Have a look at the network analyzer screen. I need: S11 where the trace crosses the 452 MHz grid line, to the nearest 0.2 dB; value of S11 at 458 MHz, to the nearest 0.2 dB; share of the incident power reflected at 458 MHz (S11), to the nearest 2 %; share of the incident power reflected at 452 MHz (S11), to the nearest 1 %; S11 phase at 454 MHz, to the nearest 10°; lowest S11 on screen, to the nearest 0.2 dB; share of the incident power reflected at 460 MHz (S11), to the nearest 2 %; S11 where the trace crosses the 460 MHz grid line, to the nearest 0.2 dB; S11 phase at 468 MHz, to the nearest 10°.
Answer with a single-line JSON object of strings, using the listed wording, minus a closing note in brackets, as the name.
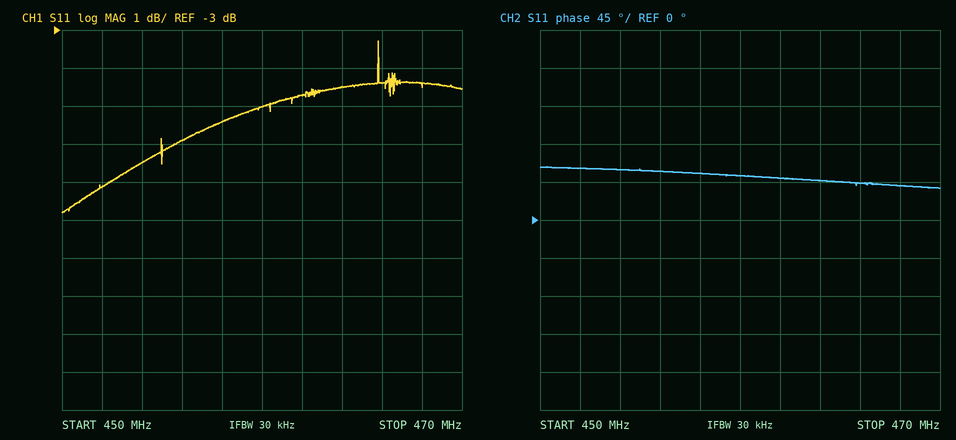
{"S11 where the trace crosses the 452 MHz grid line, to the nearest 0.2 dB": "-7.2 dB", "value of S11 at 458 MHz, to the nearest 0.2 dB": "-5.4 dB", "share of the incident power reflected at 458 MHz (S11), to the nearest 2 %": "28 %", "share of the incident power reflected at 452 MHz (S11), to the nearest 1 %": "19 %", "S11 phase at 454 MHz, to the nearest 10°": "60°", "lowest S11 on screen, to the nearest 0.2 dB": "-7.8 dB", "share of the incident power reflected at 460 MHz (S11), to the nearest 2 %": "32 %", "S11 where the trace crosses the 460 MHz grid line, to the nearest 0.2 dB": "-5.0 dB", "S11 phase at 468 MHz, to the nearest 10°": "40°"}
